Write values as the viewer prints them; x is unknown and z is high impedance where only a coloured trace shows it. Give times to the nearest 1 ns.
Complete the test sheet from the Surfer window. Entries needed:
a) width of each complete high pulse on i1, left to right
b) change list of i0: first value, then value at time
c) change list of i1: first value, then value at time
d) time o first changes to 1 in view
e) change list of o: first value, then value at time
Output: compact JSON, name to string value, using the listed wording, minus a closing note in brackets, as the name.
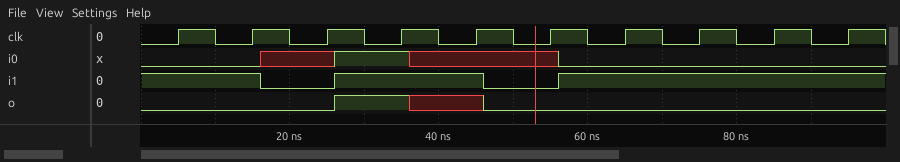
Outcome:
{"width of each complete high pulse on i1, left to right": "20 ns", "change list of i0: first value, then value at time": "0, x at 16 ns, 1 at 26 ns, x at 36 ns, 0 at 56 ns", "change list of i1: first value, then value at time": "1, 0 at 16 ns, 1 at 26 ns, 0 at 46 ns, 1 at 56 ns", "time o first changes to 1 in view": "26 ns", "change list of o: first value, then value at time": "0, 1 at 26 ns, x at 36 ns, 0 at 46 ns"}
